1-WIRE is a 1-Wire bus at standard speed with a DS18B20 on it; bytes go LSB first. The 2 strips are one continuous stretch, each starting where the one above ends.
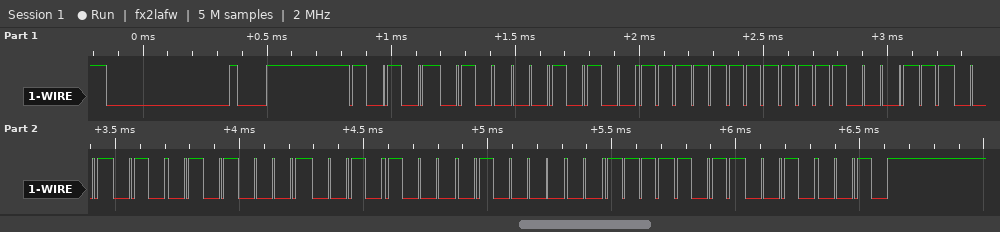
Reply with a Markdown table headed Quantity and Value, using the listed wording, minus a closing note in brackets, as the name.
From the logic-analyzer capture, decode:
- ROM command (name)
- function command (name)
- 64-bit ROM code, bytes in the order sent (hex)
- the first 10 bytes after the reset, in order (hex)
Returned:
| Quantity | Value |
|---|---|
| ROM command | Match ROM |
| function command | Convert T |
| 64-bit ROM code, bytes in the order sent | 28 FF 8F 53 8A 14 02 DF |
| the first 10 bytes after the reset, in order | 55 28 FF 8F 53 8A 14 02 DF 44 |
